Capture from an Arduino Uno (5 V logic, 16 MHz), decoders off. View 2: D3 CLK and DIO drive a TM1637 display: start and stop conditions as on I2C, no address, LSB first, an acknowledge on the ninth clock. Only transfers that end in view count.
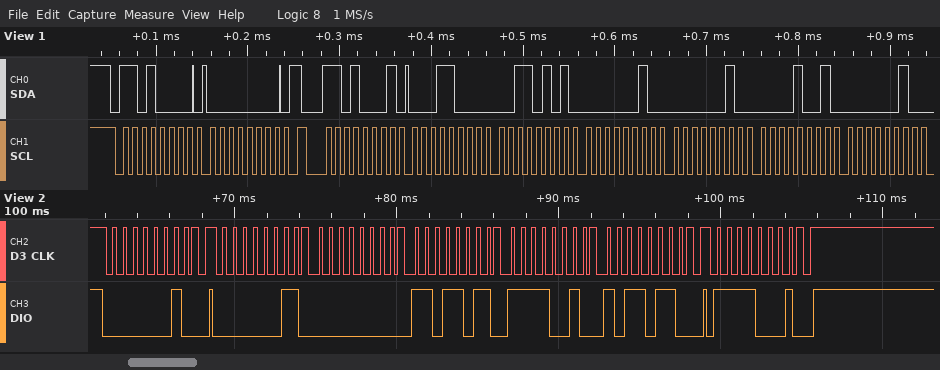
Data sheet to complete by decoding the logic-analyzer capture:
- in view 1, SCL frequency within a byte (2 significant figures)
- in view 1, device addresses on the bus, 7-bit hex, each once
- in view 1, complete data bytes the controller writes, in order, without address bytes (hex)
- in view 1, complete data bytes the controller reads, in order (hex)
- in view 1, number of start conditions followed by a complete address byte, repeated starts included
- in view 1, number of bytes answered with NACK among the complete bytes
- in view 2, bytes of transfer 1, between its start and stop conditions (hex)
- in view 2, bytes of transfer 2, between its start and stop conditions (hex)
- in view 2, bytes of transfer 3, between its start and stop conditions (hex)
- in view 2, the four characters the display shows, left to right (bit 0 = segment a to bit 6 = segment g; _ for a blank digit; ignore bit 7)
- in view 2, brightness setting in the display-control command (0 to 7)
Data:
100 kHz
0x68
00
18 35 02 02 09 02
2
0
40
C0 00 DB 4F 6D
8F
_235
7
